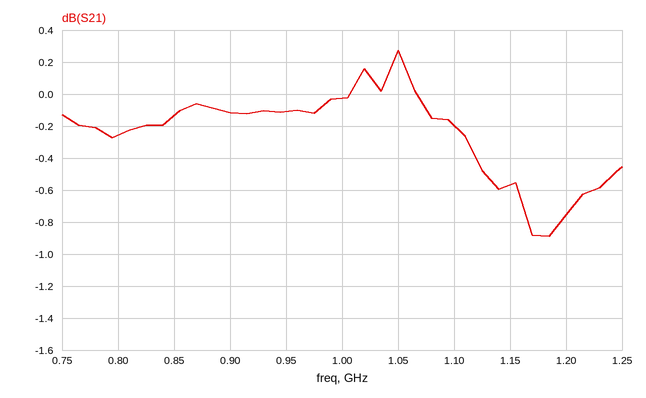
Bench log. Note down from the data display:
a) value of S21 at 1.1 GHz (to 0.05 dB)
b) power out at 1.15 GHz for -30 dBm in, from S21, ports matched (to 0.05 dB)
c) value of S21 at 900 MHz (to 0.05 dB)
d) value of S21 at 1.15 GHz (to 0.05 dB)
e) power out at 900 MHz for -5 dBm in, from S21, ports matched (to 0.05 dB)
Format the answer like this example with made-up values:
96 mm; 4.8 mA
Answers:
-0.20 dB; -30.55 dBm; -0.10 dB; -0.55 dB; -5.10 dBm
